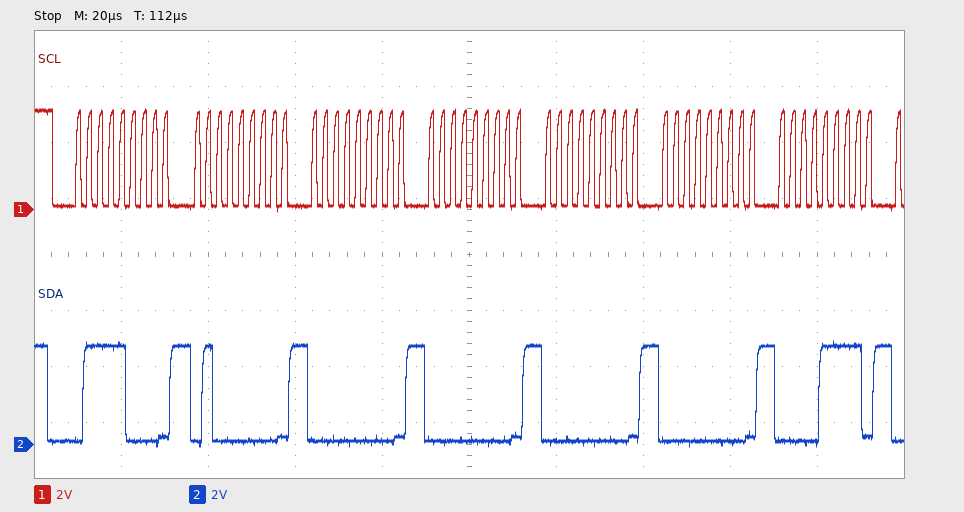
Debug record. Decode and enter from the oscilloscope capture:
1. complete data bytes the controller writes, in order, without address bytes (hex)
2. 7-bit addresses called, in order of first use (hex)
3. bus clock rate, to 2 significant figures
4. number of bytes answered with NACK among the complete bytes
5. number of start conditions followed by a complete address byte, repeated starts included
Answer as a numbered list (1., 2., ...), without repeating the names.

1. 40 00 00 00 00 0F
2. 0x3C
3. 400 kHz
4. 0
5. 1
